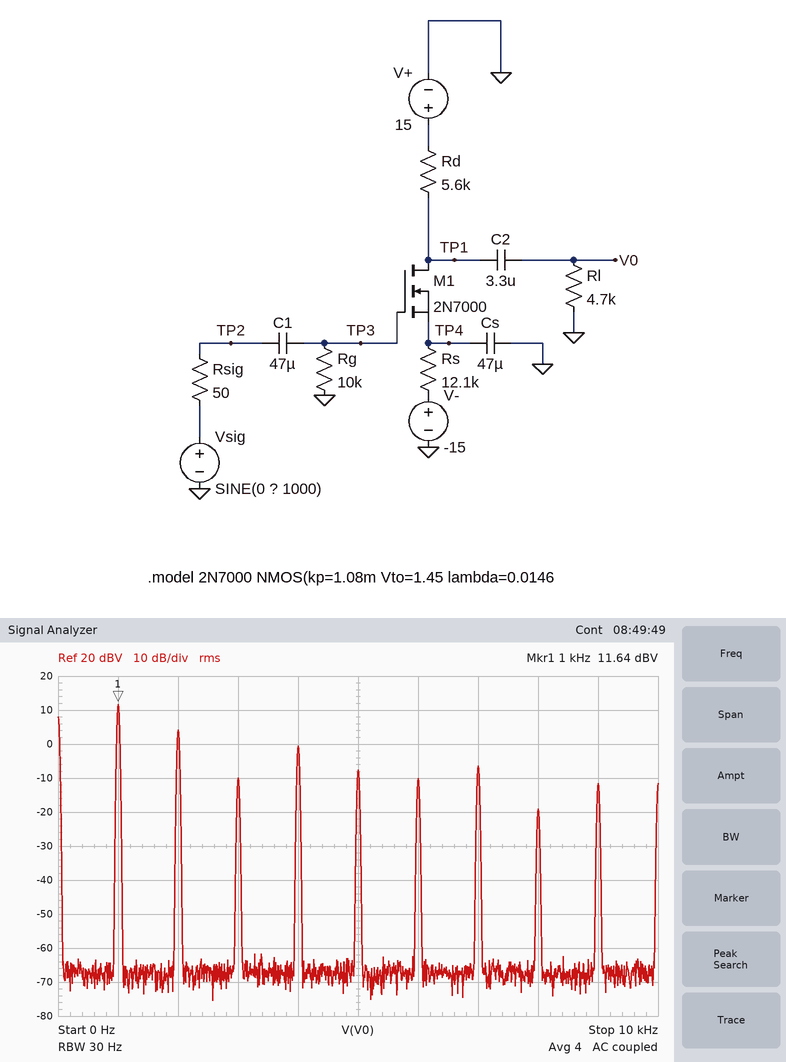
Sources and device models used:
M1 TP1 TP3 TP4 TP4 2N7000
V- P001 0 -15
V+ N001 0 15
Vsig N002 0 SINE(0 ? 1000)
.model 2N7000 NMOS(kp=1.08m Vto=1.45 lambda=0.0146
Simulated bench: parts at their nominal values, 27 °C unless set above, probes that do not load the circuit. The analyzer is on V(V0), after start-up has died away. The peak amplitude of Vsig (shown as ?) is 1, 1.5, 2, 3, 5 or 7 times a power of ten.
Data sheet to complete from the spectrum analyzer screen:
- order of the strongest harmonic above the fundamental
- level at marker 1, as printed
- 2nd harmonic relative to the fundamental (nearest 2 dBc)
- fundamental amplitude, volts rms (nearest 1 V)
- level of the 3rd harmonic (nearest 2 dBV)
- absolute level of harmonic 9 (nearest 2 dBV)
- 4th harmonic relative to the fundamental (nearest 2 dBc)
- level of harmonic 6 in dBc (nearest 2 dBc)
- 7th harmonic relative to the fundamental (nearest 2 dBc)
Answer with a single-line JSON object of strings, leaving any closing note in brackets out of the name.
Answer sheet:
{"order of the strongest harmonic above the fundamental": "2", "level at marker 1, as printed": "11.64 dBV", "2nd harmonic relative to the fundamental": "-8 dBc", "fundamental amplitude, volts rms": "4 V", "level of the 3rd harmonic": "-10 dBV", "absolute level of harmonic 9": "-12 dBV", "4th harmonic relative to the fundamental": "-12 dBc", "level of harmonic 6 in dBc": "-22 dBc", "7th harmonic relative to the fundamental": "-18 dBc"}
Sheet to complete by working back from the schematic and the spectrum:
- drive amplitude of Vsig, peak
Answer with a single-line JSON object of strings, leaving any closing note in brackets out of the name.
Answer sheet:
{"drive amplitude of Vsig, peak": "10 V"}
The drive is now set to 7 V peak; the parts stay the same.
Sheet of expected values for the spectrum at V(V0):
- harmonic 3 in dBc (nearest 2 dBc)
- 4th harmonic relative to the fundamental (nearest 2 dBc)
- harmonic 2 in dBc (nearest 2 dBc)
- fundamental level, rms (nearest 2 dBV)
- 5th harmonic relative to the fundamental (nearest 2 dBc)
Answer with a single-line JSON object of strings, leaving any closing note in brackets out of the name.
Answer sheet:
{"harmonic 3 in dBc": "-32 dBc", "4th harmonic relative to the fundamental": "-14 dBc", "harmonic 2 in dBc": "-6 dBc", "fundamental level, rms": "12 dBV", "5th harmonic relative to the fundamental": "-16 dBc"}
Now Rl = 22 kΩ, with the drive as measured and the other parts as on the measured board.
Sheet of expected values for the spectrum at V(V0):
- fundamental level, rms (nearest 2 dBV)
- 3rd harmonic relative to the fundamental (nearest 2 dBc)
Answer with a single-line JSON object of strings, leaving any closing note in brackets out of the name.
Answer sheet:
{"fundamental level, rms": "16 dBV", "3rd harmonic relative to the fundamental": "-14 dBc"}
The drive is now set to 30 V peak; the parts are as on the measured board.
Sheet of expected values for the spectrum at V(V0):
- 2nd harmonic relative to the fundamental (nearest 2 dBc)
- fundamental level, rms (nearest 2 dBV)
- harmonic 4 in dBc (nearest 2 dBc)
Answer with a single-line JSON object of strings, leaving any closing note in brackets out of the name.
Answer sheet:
{"2nd harmonic relative to the fundamental": "-14 dBc", "fundamental level, rms": "12 dBV", "harmonic 4 in dBc": "-16 dBc"}
